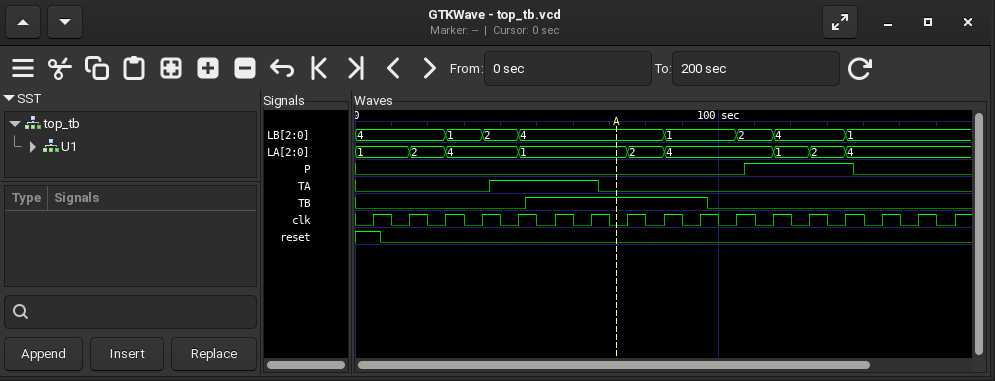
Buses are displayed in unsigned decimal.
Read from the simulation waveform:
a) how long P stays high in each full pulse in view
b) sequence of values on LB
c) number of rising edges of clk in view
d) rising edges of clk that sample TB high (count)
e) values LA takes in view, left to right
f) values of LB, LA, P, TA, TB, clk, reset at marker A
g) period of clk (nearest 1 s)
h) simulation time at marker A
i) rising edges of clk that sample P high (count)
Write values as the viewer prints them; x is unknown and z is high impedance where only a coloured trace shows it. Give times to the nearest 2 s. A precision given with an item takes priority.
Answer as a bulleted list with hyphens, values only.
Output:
- 30 s
- 4, 1, 2, 4, 1, 2, 4, 1
- 17
- 5
- 1, 2, 4, 1, 2, 4, 1, 2, 4
- LB=4, LA=1, P=0, TA=0, TB=1, clk=0, reset=0
- 10 s
- 72 s
- 3
